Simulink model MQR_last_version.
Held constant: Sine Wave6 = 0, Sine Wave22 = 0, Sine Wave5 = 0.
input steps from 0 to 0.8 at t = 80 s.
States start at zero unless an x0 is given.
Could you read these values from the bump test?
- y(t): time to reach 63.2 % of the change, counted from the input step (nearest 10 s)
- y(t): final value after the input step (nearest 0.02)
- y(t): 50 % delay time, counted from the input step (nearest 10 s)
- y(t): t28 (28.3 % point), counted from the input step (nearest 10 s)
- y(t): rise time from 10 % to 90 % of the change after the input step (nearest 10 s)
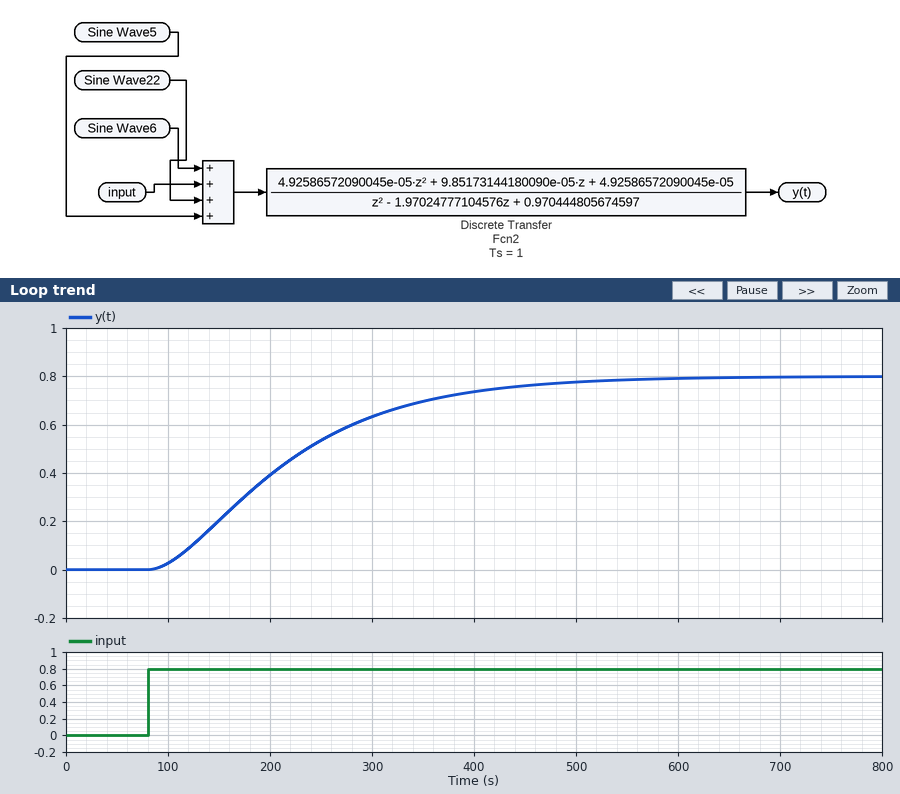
160 s
0.80
120 s
80 s
260 s
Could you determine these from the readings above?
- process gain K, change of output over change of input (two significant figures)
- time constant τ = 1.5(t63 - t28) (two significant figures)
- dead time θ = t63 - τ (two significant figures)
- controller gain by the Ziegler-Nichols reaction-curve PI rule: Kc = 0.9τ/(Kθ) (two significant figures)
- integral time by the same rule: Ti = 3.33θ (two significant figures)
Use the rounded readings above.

1.0
120 s
40 s
2.7
130 s
